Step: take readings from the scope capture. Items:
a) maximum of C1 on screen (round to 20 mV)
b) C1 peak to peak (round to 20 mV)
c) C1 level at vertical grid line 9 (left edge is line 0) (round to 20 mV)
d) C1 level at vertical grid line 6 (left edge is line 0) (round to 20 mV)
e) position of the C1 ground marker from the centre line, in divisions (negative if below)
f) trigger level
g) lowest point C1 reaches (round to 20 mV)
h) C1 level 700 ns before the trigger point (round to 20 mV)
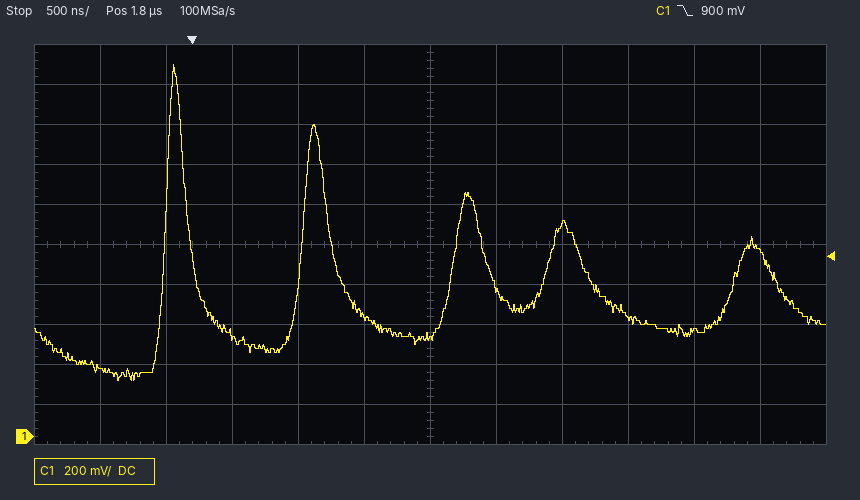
1.86 V
1.58 V
600 mV
500 mV
-4.8 div
900 mV
280 mV
340 mV
